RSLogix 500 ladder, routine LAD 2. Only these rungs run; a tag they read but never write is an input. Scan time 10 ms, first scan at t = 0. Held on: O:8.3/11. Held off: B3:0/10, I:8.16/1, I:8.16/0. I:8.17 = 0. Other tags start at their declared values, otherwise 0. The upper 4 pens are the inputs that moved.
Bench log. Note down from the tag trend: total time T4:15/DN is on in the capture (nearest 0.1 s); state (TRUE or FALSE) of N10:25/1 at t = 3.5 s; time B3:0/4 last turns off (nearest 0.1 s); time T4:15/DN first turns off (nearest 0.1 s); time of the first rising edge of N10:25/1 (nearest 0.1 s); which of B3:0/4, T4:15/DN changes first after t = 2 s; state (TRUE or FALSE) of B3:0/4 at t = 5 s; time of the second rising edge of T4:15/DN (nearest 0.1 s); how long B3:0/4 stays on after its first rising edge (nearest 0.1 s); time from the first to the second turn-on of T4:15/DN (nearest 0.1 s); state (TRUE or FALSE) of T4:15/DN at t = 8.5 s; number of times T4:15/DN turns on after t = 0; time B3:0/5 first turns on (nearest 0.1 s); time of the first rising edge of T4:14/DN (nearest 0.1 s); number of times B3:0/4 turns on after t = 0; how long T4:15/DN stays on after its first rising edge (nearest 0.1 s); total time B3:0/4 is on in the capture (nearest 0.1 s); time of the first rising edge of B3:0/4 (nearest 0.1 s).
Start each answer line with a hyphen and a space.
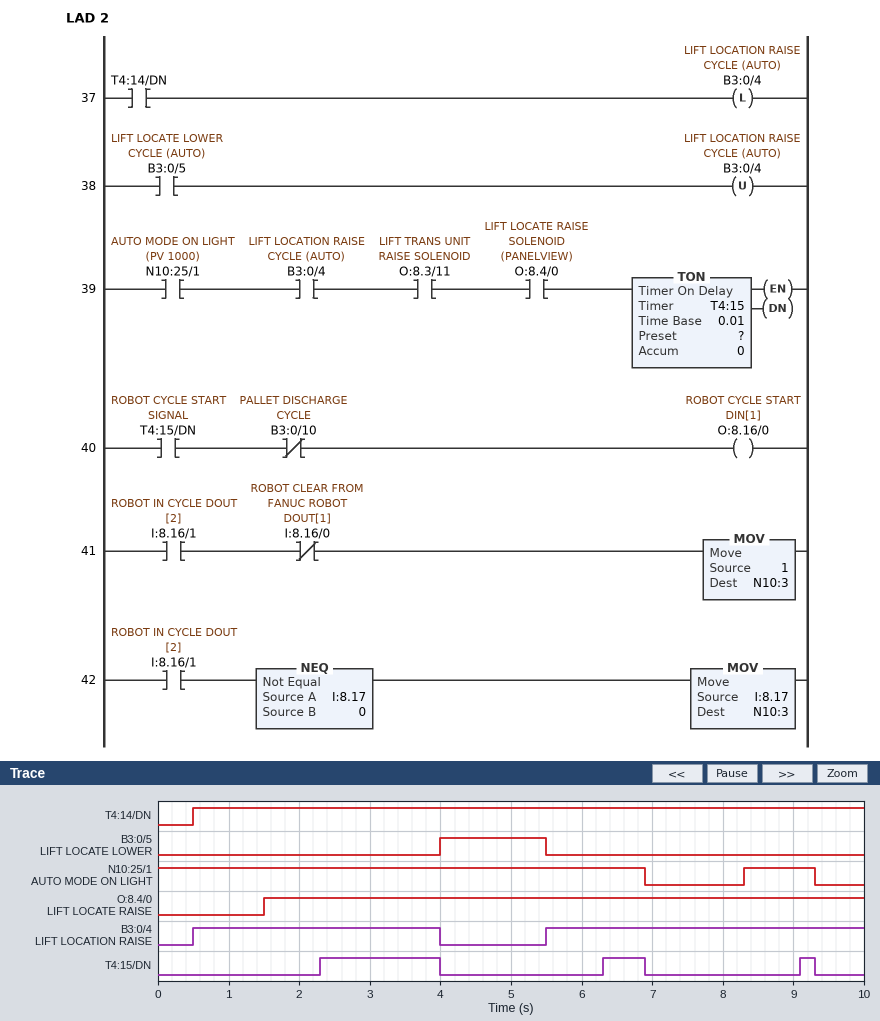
- 2.5 s
- TRUE
- 4.0 s
- 4.0 s
- 8.3 s
- T4:15/DN
- FALSE
- 6.3 s
- 3.5 s
- 4.0 s
- FALSE
- 3
- 4.0 s
- 0.5 s
- 2
- 1.7 s
- 8.0 s
- 0.5 s
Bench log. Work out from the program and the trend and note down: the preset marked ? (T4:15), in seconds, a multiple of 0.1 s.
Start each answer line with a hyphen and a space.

- 0.8 s
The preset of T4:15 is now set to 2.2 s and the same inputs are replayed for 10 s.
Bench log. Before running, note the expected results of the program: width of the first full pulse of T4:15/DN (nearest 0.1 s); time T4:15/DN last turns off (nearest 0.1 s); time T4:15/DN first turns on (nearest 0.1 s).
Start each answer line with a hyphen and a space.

- 0.3 s
- 4.0 s
- 3.7 s
